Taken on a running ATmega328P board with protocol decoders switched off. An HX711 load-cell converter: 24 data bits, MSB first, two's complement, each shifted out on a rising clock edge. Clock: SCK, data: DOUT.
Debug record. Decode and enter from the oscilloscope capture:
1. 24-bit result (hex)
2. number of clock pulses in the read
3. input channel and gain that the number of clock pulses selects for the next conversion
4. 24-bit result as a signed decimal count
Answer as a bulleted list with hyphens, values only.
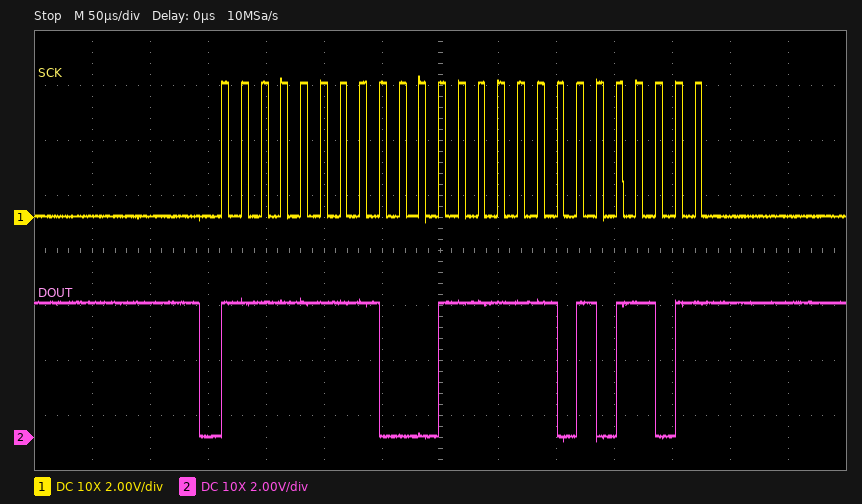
- 0xFF1FAD
- 25
- channel A, gain 128
- -57427
